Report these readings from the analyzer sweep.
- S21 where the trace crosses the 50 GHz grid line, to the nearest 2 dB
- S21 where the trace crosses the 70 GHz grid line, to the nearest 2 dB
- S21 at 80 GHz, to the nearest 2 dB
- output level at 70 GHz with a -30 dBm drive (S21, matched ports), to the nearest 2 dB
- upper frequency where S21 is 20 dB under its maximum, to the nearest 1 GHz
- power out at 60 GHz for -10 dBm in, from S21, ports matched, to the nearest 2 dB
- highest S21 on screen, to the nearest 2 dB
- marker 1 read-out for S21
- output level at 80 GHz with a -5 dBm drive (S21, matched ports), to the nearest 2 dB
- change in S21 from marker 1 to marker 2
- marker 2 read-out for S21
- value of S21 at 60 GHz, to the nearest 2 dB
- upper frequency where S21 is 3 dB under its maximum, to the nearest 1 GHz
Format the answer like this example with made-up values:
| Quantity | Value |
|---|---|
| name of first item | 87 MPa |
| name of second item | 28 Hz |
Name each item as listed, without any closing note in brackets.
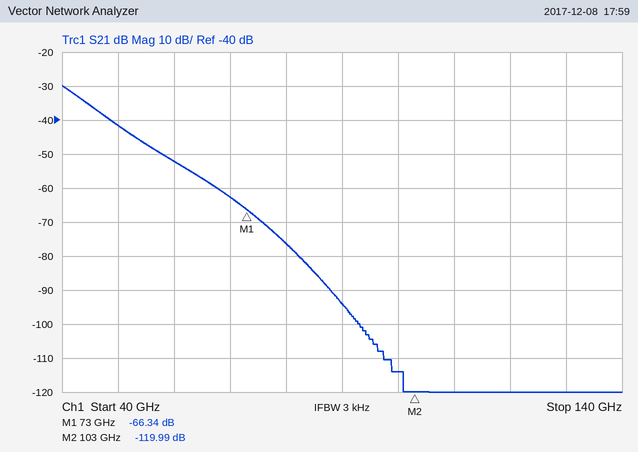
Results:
| Quantity | Value |
|---|---|
| S21 where the trace crosses the 50 GHz grid line, to the nearest 2 dB | -42 dB |
| S21 where the trace crosses the 70 GHz grid line, to the nearest 2 dB | -62 dB |
| S21 at 80 GHz, to the nearest 2 dB | -76 dB |
| output level at 70 GHz with a -30 dBm drive (S21, matched ports), to the nearest 2 dB | -92 dBm |
| upper frequency where S21 is 20 dB under its maximum, to the nearest 1 GHz | 58 GHz |
| power out at 60 GHz for -10 dBm in, from S21, ports matched, to the nearest 2 dB | -62 dBm |
| highest S21 on screen, to the nearest 2 dB | -30 dB |
| marker 1 read-out for S21 | -66.34 dB |
| output level at 80 GHz with a -5 dBm drive (S21, matched ports), to the nearest 2 dB | -82 dBm |
| change in S21 from marker 1 to marker 2 | -53.65 dB |
| marker 2 read-out for S21 | -119.99 dB |
| value of S21 at 60 GHz, to the nearest 2 dB | -52 dB |
| upper frequency where S21 is 3 dB under its maximum, to the nearest 1 GHz | 43 GHz |
